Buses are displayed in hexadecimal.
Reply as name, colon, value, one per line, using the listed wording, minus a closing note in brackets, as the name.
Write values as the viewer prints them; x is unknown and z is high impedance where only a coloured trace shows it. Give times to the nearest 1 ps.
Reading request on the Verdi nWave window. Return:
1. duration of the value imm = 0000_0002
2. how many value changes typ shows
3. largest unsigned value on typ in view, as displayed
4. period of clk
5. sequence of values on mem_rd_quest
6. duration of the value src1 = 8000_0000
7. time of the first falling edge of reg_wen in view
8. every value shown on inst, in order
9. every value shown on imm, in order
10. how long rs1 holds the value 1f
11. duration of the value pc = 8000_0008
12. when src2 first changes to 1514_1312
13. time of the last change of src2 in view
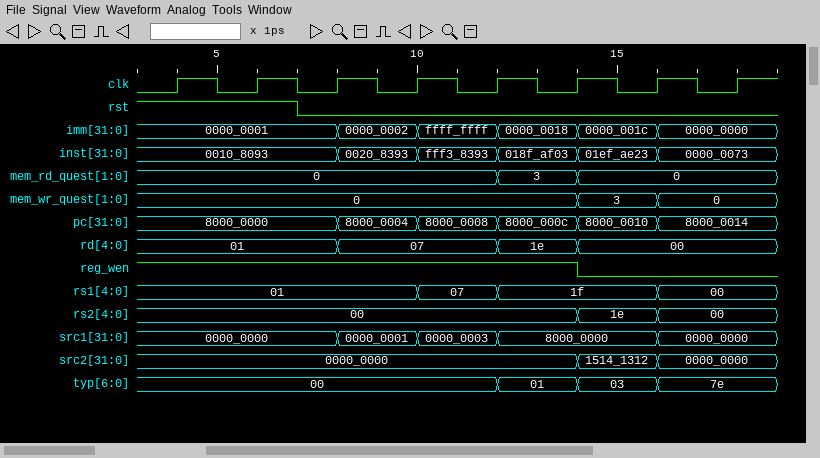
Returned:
duration of the value imm = 0000_0002: 2 ps
how many value changes typ shows: 3
largest unsigned value on typ in view, as displayed: 7e
period of clk: 2 ps
sequence of values on mem_rd_quest: 0, 3, 0
duration of the value src1 = 8000_0000: 4 ps
time of the first falling edge of reg_wen in view: 14 ps
every value shown on inst, in order: 0010_8093, 0020_8393, fff3_8393, 018f_af03, 01ef_ae23, 0000_0073
every value shown on imm, in order: 0000_0001, 0000_0002, ffff_ffff, 0000_0018, 0000_001c, 0000_0000
how long rs1 holds the value 1f: 4 ps
duration of the value pc = 8000_0008: 2 ps
when src2 first changes to 1514_1312: 14 ps
time of the last change of src2 in view: 16 ps
